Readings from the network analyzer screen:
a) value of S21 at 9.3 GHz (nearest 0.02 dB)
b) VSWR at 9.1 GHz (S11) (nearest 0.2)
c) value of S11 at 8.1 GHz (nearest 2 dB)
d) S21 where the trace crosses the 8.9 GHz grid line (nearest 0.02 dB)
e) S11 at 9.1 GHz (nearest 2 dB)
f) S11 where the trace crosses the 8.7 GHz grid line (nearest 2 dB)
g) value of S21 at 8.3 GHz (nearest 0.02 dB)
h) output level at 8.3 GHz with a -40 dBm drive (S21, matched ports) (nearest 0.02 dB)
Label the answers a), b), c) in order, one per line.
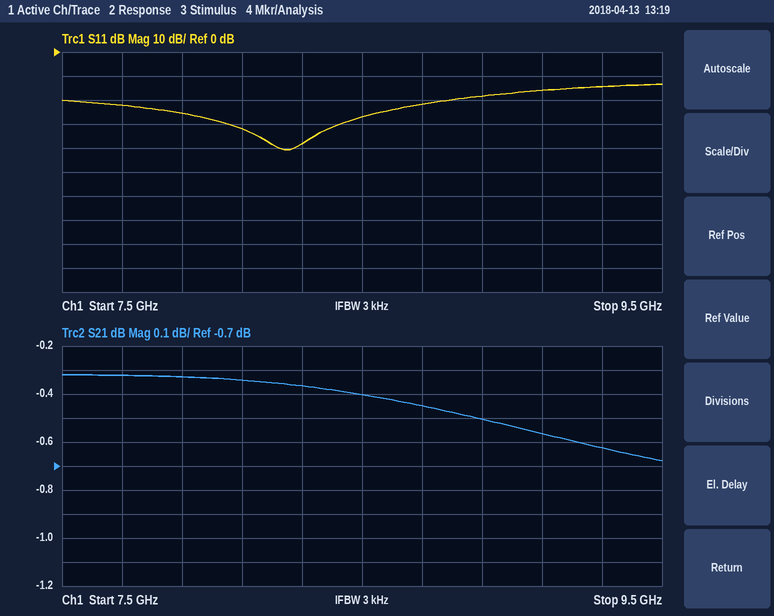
a) -0.62 dB
b) 1.4
c) -32 dB
d) -0.50 dB
e) -16 dB
f) -22 dB
g) -0.36 dB
h) -40.36 dBm
